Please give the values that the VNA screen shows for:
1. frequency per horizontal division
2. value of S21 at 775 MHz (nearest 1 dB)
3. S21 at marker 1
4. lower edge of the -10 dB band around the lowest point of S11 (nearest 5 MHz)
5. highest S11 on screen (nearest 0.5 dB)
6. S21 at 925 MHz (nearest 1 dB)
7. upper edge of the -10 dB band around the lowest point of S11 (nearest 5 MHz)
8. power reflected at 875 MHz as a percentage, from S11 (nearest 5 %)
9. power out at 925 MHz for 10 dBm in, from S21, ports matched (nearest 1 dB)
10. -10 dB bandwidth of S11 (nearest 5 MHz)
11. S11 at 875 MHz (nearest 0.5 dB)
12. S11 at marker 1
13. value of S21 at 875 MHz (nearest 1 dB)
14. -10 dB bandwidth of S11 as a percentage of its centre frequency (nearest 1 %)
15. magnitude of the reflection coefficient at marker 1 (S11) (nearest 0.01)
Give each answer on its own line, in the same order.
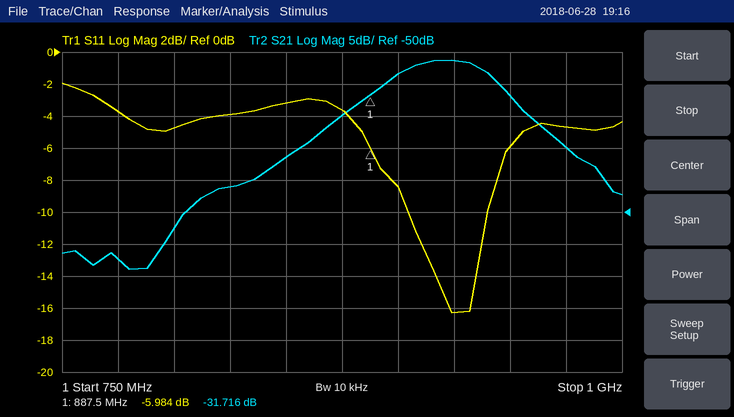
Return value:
25 MHz
-57 dB
-31.716 dB
905 MHz
-2.0 dB
-26 dB
940 MHz
45 %
-16 dBm
35 MHz
-3.5 dB
-5.984 dB
-35 dB
4 %
0.50
